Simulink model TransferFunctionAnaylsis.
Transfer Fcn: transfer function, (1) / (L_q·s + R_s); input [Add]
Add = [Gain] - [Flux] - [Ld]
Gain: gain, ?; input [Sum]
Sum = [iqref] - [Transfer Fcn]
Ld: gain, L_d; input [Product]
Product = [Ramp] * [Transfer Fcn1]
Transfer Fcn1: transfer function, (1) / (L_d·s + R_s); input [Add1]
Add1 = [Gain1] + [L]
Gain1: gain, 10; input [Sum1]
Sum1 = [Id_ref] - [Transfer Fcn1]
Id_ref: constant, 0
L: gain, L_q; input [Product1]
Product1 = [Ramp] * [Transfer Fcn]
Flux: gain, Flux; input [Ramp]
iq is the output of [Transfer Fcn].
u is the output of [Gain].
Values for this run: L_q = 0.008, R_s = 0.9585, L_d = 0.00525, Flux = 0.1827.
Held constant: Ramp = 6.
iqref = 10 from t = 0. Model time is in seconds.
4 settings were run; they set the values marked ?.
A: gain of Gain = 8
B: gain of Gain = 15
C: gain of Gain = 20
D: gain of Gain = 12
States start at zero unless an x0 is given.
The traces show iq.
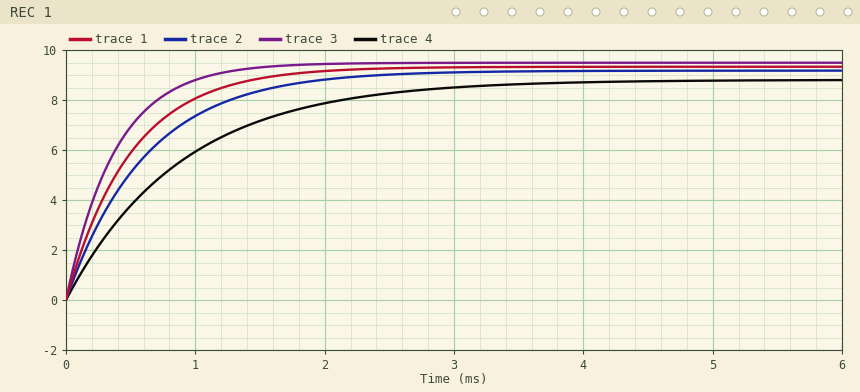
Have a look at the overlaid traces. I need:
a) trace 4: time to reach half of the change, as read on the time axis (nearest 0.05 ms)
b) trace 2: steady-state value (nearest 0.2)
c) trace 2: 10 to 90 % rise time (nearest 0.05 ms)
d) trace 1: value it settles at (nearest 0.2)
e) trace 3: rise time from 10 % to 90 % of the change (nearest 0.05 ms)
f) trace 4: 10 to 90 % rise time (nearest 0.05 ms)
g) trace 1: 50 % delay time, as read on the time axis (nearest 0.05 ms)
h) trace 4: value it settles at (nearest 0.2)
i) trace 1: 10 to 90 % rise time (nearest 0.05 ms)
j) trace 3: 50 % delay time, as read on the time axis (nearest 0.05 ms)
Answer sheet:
0.60 ms
9.2
1.35 ms
9.4
0.85 ms
1.95 ms
0.35 ms
8.8
1.10 ms
0.25 ms
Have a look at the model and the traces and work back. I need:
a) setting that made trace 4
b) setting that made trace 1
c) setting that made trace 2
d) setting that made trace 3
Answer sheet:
A
B
D
C
